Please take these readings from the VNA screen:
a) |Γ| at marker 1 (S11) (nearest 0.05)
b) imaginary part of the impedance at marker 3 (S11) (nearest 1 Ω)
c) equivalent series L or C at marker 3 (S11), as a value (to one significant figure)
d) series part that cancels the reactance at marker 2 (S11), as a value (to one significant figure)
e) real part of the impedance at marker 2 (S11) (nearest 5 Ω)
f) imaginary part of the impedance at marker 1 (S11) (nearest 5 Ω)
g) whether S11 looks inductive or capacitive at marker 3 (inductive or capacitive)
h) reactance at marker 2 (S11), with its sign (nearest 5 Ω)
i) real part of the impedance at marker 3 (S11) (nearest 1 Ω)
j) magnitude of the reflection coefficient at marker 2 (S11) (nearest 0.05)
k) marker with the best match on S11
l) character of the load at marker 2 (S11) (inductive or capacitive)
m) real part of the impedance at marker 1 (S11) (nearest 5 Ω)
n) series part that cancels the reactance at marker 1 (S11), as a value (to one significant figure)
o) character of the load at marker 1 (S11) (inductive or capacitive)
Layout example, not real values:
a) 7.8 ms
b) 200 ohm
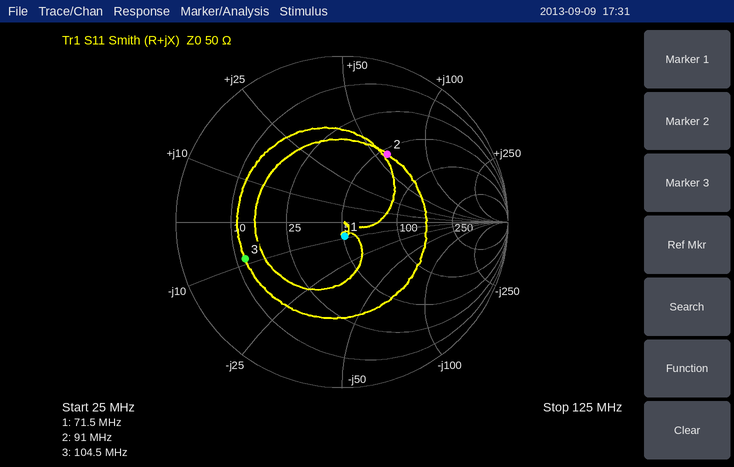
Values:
a) 0.10
b) -9 Ω
c) 200 pF
d) 30 pF
e) 55 Ω
f) -10 Ω
g) capacitive
h) +60 Ω
i) 12 Ω
j) 0.50
k) marker 1
l) inductive
m) 50 Ω
n) 20 nH
o) capacitive
